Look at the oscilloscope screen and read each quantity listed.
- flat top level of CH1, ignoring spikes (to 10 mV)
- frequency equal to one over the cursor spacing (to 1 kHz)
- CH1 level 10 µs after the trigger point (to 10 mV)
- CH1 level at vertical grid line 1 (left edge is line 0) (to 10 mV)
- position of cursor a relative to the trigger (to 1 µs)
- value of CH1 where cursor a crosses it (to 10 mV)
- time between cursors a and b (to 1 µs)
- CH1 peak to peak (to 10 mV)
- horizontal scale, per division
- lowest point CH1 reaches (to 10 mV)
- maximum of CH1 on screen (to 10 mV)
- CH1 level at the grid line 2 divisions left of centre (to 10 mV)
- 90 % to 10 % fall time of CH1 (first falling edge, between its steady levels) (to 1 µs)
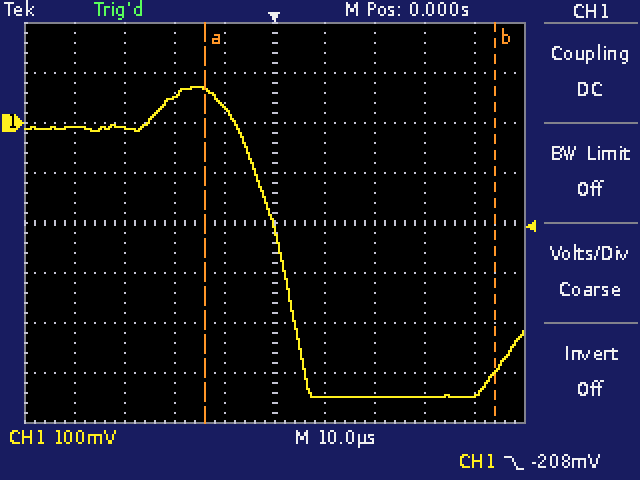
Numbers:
-10 mV
17 kHz
-550 mV
-10 mV
-14 µs
70 mV
58 µs
620 mV
10 µs
-550 mV
70 mV
50 mV
11 µs
